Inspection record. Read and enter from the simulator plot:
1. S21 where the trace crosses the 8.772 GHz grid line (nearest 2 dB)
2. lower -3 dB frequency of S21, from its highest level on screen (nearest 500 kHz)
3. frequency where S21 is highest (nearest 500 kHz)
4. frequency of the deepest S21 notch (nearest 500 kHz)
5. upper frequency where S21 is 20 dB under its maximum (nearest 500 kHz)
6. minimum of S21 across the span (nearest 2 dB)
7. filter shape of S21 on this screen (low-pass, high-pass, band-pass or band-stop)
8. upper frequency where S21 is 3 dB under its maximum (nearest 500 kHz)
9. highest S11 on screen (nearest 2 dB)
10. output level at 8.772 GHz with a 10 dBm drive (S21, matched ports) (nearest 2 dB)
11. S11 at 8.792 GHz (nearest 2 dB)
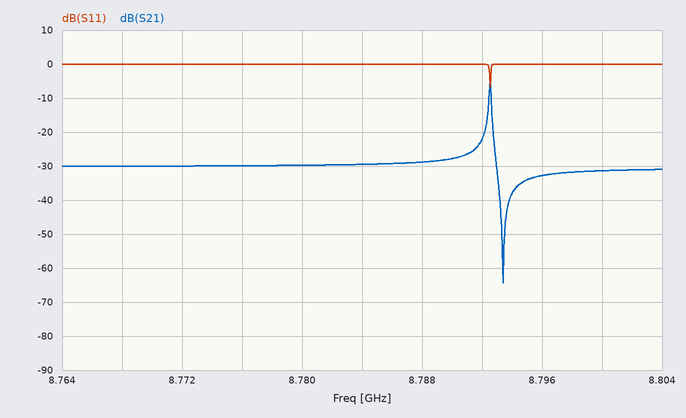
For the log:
-30 dB
8.7925 GHz
8.7925 GHz
8.7935 GHz
8.7930 GHz
-64 dB
band-pass
8.7925 GHz
0 dB
-20 dBm
0 dB
